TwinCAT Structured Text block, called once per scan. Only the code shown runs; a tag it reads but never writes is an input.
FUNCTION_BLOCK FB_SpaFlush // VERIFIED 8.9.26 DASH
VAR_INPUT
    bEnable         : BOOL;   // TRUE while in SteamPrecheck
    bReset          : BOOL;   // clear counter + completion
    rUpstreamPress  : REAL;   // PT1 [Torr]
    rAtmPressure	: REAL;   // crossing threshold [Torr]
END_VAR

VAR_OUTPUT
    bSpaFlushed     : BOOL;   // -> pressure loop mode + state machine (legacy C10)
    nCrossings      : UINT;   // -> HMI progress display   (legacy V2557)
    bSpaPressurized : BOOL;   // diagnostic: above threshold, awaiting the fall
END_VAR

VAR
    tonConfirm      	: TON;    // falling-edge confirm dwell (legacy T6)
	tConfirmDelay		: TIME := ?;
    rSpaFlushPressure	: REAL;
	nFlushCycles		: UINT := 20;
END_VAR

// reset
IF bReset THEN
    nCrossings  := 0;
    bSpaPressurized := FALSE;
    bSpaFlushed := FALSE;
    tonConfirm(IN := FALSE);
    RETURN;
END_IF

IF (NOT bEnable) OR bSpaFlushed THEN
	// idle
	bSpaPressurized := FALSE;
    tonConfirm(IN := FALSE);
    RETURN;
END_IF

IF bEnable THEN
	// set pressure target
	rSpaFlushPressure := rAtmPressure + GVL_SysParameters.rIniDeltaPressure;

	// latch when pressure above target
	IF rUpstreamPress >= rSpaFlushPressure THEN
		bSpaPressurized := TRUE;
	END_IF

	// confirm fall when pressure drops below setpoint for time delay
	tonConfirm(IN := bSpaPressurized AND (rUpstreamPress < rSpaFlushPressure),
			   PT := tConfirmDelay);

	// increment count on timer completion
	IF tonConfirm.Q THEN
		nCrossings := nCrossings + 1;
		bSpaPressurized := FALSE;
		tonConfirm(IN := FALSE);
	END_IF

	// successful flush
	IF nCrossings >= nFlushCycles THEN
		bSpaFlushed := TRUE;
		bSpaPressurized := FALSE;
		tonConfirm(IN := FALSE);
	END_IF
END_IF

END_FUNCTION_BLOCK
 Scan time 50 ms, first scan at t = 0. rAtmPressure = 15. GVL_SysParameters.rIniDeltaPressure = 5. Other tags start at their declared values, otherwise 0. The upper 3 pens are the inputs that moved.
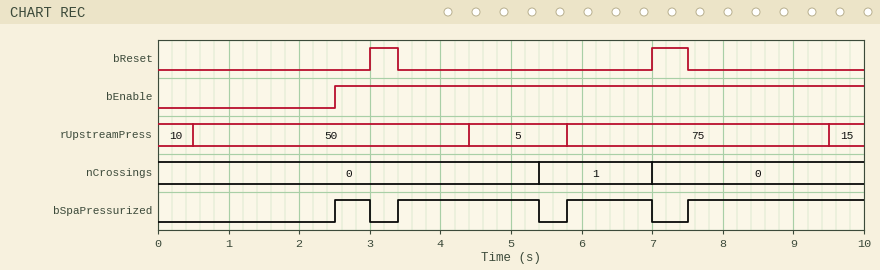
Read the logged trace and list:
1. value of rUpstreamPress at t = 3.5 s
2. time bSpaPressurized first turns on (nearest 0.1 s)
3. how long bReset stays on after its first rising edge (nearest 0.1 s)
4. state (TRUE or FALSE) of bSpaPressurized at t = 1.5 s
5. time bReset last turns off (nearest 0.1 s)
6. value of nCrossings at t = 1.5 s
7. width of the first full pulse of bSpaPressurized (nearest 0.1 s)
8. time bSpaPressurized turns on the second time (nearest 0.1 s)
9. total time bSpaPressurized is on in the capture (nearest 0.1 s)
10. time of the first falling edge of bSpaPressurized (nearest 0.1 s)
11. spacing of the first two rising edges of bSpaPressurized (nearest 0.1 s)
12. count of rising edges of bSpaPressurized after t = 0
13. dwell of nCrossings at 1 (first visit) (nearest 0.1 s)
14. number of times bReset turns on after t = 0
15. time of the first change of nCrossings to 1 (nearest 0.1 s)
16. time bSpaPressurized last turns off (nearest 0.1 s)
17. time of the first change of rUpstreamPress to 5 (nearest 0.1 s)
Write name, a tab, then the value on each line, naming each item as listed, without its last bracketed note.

value of rUpstreamPress at t = 3.5 s	50
time bSpaPressurized first turns on	2.5 s
how long bReset stays on after its first rising edge	0.4 s
state (TRUE or FALSE) of bSpaPressurized at t = 1.5 s	FALSE
time bReset last turns off	7.5 s
value of nCrossings at t = 1.5 s	0
width of the first full pulse of bSpaPressurized	0.5 s
time bSpaPressurized turns on the second time	3.4 s
total time bSpaPressurized is on in the capture	6.2 s
time of the first falling edge of bSpaPressurized	3.0 s
spacing of the first two rising edges of bSpaPressurized	0.9 s
count of rising edges of bSpaPressurized after t = 0	4
dwell of nCrossings at 1 (first visit)	1.6 s
number of times bReset turns on after t = 0	2
time of the first change of nCrossings to 1	5.4 s
time bSpaPressurized last turns off	7.0 s
time of the first change of rUpstreamPress to 5	4.4 s
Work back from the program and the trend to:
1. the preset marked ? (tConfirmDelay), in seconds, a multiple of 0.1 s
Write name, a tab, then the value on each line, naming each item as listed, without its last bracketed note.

the preset marked ? (tConfirmDelay), in seconds, a multiple of 0.1 s	1.0 s
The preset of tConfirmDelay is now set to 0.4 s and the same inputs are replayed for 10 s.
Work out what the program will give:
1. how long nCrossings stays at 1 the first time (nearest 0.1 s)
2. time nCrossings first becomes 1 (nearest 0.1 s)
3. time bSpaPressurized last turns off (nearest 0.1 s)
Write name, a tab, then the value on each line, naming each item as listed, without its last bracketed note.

how long nCrossings stays at 1 the first time	2.2 s
time nCrossings first becomes 1	4.8 s
time bSpaPressurized last turns off	9.9 s
